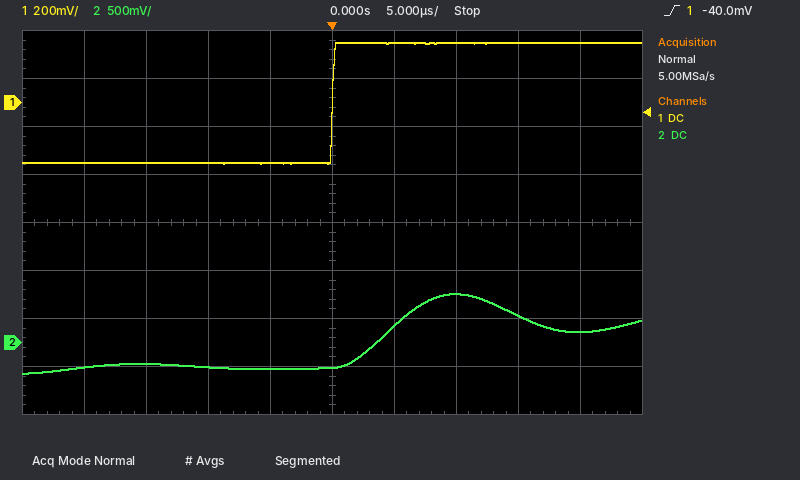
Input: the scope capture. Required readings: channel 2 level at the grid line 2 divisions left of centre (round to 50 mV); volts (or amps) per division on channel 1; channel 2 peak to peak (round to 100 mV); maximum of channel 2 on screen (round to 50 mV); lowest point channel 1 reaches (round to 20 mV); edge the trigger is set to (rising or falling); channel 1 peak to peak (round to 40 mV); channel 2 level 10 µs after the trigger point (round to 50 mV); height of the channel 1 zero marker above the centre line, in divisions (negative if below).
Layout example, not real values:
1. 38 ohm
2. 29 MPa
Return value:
1. -250 mV
2. 200 mV
3. 800 mV
4. 500 mV
5. -260 mV
6. rising
7. 520 mV
8. 500 mV
9. +2.5 div
